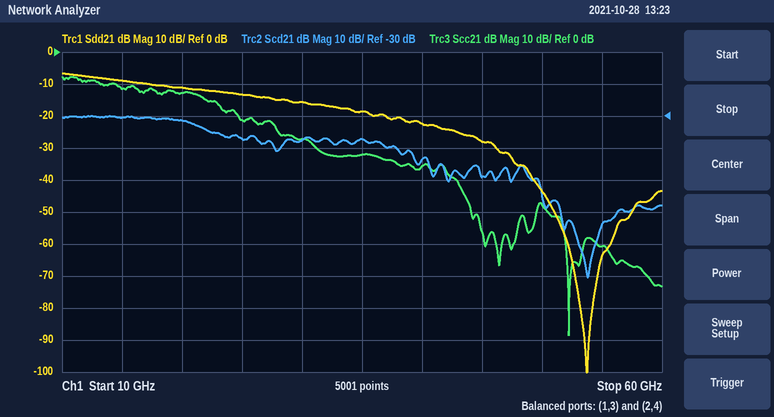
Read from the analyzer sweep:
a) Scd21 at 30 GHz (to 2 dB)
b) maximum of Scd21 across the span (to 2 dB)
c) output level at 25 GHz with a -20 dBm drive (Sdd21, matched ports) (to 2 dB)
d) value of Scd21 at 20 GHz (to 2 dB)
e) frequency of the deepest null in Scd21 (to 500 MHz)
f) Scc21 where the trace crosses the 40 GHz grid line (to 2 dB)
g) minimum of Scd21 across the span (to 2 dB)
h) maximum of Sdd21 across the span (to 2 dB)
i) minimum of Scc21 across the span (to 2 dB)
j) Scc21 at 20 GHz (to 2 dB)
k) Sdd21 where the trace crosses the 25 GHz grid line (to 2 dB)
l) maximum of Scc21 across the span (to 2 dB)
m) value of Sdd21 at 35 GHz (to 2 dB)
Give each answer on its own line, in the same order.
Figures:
-38 dB
-30 dB
-34 dBm
-32 dB
54.0 GHz
-36 dB
-80 dB
-6 dB
-88 dB
-12 dB
-14 dB
-8 dB
-18 dB
